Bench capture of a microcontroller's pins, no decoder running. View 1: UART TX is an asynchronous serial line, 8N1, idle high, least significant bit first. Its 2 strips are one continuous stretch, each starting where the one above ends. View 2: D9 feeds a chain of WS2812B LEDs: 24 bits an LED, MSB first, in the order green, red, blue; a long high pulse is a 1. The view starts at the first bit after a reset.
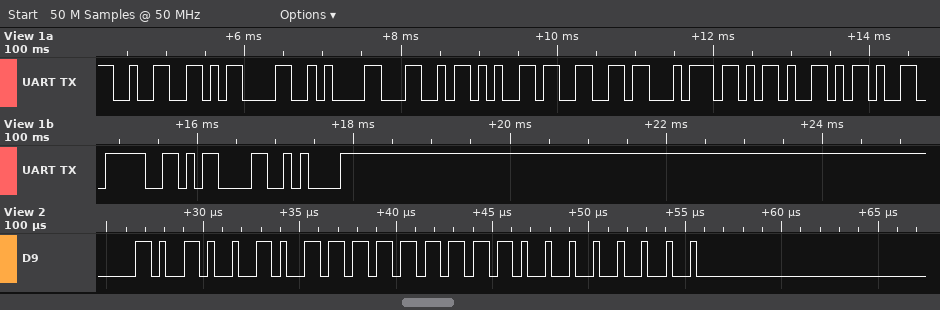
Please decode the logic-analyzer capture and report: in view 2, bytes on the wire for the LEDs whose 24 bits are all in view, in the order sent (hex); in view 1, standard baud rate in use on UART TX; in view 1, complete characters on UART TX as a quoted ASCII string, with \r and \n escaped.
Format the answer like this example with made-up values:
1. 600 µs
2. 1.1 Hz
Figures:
1. A5 FF 00
2. 9600 baud
3. "2\r\nLeft-->\r\n"
